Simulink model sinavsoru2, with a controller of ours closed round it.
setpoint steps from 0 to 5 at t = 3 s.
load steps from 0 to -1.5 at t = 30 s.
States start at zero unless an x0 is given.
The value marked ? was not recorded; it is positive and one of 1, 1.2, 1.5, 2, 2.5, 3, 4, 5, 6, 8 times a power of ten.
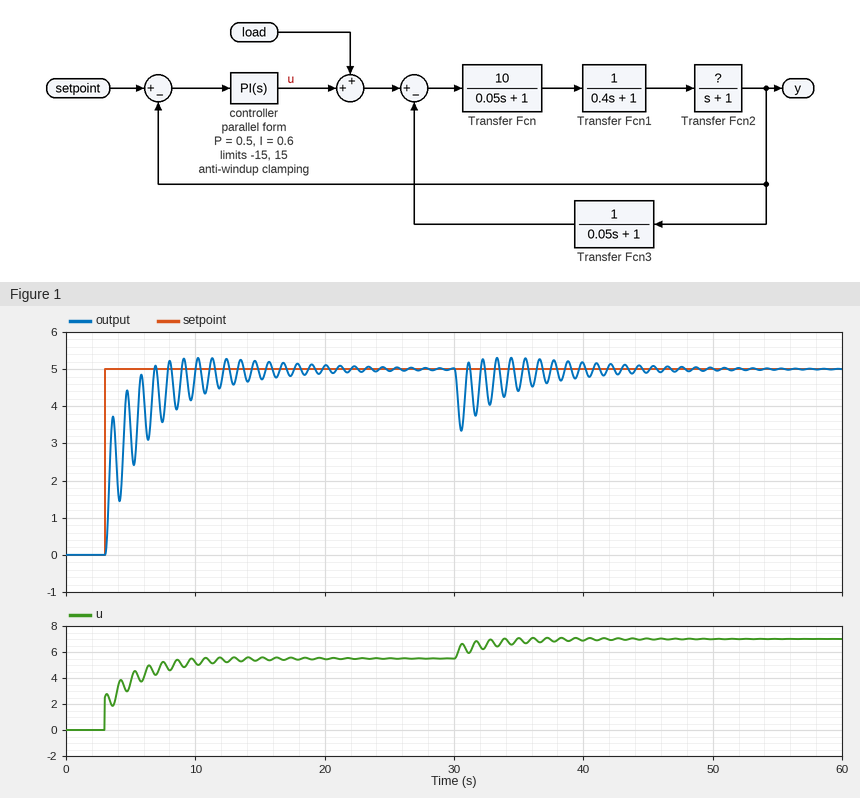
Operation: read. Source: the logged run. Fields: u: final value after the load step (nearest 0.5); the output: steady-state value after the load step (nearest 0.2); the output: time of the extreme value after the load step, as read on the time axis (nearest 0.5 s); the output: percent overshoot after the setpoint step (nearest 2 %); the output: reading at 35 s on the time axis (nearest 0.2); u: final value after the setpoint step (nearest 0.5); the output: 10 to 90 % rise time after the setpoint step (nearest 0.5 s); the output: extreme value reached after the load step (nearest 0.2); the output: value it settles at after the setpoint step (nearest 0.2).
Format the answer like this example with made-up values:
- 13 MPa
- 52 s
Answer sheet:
- 7.0
- 5.0
- 30.5 s
- 6 %
- 4.4
- 5.5
- 2.5 s
- 3.4
- 5.0
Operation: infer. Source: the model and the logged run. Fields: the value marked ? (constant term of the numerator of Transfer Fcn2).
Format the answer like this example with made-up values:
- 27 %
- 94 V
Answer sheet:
- 1
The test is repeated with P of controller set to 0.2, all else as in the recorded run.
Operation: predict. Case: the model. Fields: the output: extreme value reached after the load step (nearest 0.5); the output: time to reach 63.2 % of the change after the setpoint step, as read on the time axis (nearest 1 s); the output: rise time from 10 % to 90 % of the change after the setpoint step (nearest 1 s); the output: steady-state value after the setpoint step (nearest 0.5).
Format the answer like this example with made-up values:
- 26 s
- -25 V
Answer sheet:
- 3.0
- 5 s
- 4 s
- 5.0
